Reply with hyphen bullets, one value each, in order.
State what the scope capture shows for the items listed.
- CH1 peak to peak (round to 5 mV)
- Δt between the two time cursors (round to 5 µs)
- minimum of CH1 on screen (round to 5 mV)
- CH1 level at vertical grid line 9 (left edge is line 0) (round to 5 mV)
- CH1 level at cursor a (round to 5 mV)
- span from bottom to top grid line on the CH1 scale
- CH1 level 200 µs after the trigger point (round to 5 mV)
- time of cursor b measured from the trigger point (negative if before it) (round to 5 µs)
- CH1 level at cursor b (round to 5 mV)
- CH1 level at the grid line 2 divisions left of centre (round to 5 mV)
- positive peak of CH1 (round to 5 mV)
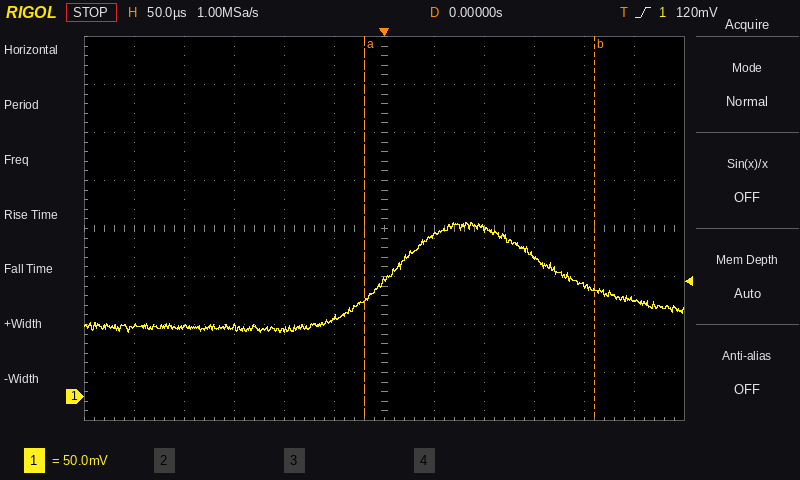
- 115 mV
- 230 µs
- 65 mV
- 145 mV
- 100 mV
- 400 mV
- 115 mV
- +210 µs
- 110 mV
- 70 mV
- 180 mV
